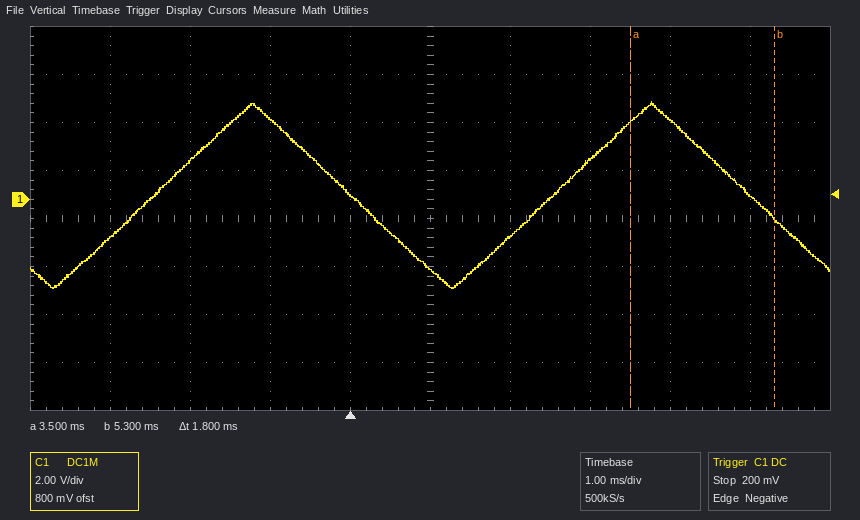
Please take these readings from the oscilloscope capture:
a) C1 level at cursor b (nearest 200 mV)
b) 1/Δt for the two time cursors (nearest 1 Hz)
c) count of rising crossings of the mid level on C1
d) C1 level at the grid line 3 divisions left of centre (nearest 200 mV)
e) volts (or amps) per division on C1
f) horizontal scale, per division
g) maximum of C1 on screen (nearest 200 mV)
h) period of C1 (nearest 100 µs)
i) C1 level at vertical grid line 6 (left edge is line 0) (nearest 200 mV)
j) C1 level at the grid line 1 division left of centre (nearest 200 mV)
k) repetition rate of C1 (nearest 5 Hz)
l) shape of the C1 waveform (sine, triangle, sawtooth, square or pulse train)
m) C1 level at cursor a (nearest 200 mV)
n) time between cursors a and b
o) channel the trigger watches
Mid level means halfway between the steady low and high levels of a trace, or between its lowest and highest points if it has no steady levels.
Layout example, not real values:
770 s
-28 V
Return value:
-800 mV
556 Hz
2
1.6 V
2 V
1 ms
4.0 V
5.0 ms
-1.6 V
200 mV
200 Hz
triangle
3.2 V
1.8 ms
C1
